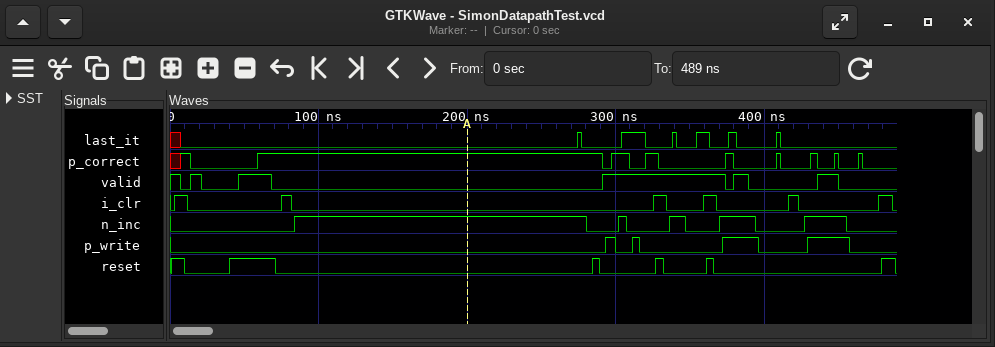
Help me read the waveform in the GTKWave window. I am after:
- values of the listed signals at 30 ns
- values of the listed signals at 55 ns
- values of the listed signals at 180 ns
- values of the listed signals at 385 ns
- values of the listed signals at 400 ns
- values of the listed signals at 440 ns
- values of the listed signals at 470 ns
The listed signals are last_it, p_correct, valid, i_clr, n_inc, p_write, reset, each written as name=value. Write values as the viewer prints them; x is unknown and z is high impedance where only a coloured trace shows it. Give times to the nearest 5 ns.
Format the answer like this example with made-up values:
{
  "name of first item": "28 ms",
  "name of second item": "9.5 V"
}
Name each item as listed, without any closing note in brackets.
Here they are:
{
  "values of the listed signals at 30 ns": "last_it=0, p_correct=0, valid=0, i_clr=0, n_inc=0, p_write=0, reset=0",
  "values of the listed signals at 55 ns": "last_it=0, p_correct=0, valid=1, i_clr=0, n_inc=0, p_write=0, reset=1",
  "values of the listed signals at 180 ns": "last_it=0, p_correct=1, valid=0, i_clr=0, n_inc=1, p_write=0, reset=0",
  "values of the listed signals at 385 ns": "last_it=0, p_correct=0, valid=1, i_clr=0, n_inc=1, p_write=1, reset=0",
  "values of the listed signals at 400 ns": "last_it=0, p_correct=0, valid=0, i_clr=0, n_inc=0, p_write=0, reset=0",
  "values of the listed signals at 440 ns": "last_it=0, p_correct=0, valid=1, i_clr=0, n_inc=1, p_write=1, reset=0",
  "values of the listed signals at 470 ns": "last_it=0, p_correct=0, valid=0, i_clr=0, n_inc=0, p_write=0, reset=0"
}
